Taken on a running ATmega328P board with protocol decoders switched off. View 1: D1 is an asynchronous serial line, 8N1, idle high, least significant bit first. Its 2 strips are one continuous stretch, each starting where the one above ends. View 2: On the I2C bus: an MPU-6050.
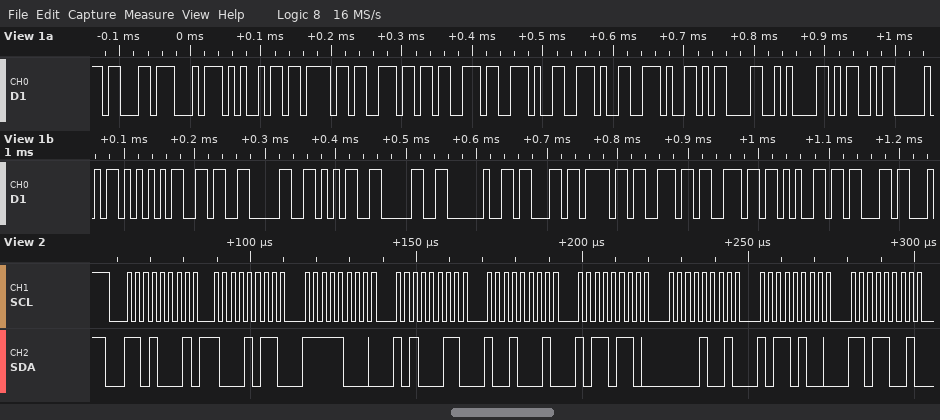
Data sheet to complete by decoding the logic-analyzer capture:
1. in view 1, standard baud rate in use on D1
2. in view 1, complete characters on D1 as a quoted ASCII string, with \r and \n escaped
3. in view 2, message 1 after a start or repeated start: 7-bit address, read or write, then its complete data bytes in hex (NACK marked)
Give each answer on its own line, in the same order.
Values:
115200 baud
"ctions...\r\nMPU6050 connec"
0x68 read: 8B F8 A3 91 B6 09 B4 D9
